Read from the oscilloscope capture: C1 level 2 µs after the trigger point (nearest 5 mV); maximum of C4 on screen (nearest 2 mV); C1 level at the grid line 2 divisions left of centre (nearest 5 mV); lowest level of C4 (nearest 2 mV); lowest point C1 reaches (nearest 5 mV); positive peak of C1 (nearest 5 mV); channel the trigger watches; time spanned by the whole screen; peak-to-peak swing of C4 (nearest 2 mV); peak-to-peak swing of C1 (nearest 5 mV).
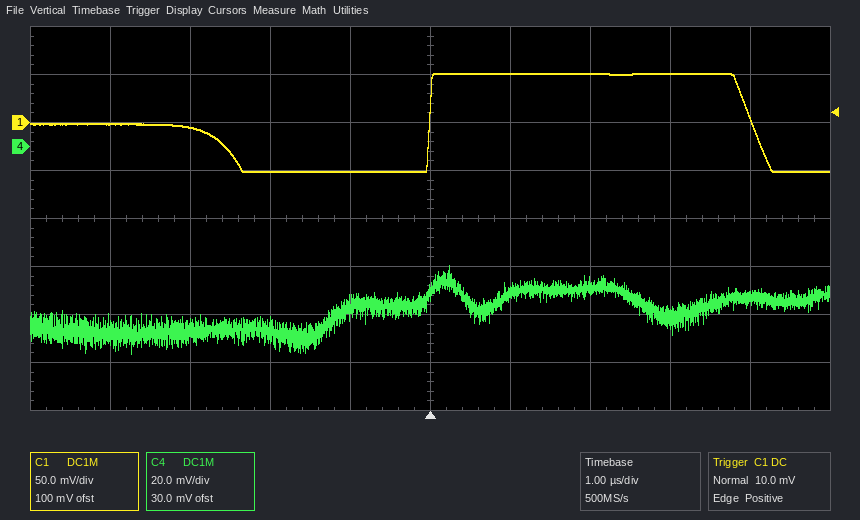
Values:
50 mV
-50 mV
-50 mV
-86 mV
-50 mV
50 mV
C1
10 µs
36 mV
100 mV
